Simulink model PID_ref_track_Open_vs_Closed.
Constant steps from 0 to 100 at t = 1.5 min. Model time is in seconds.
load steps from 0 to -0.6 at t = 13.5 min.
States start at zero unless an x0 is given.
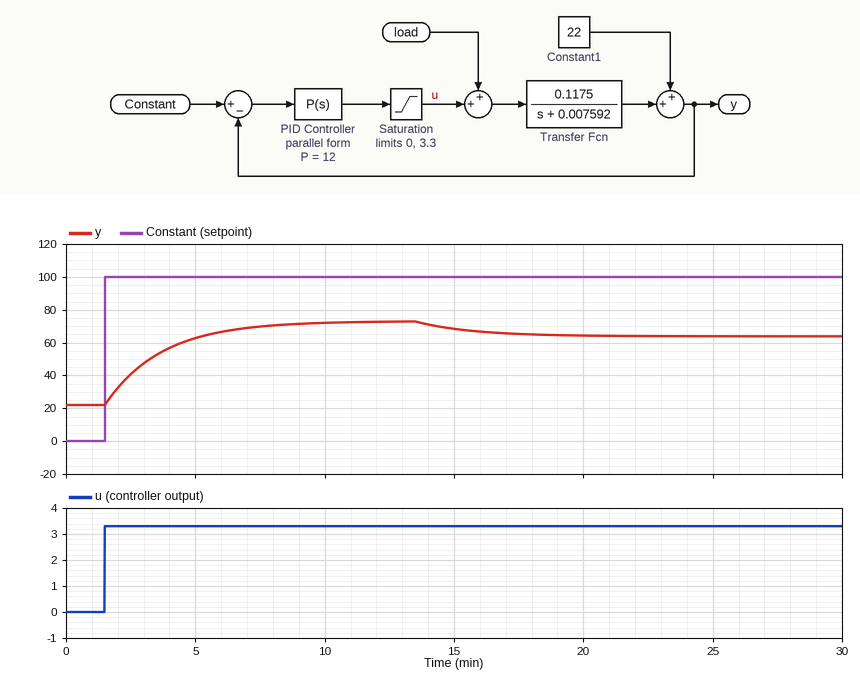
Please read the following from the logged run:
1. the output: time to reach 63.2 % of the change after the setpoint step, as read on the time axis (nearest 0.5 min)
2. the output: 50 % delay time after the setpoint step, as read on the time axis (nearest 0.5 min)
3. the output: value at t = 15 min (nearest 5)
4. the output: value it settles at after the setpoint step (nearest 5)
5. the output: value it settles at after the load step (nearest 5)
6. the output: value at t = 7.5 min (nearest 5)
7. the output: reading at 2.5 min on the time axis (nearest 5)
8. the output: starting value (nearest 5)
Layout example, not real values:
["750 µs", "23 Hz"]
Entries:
["3.5 min", "3.0 min", "70", "75", "65", "70", "40", "20"]
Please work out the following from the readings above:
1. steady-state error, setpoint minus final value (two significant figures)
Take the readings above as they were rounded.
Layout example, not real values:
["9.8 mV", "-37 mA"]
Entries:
["25"]
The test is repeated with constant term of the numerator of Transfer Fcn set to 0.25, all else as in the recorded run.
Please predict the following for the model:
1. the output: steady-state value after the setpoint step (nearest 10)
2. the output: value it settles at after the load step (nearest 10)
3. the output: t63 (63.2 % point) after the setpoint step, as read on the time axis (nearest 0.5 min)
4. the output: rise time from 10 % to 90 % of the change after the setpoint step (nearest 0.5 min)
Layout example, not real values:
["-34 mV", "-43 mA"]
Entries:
["100", "100", "3.0 min", "2.0 min"]
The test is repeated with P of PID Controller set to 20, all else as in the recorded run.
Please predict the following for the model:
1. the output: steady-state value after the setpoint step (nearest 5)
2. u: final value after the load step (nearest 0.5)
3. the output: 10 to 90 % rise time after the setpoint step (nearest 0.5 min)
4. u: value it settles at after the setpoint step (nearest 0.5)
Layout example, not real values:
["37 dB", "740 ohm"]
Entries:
["75", "3.5", "5.0 min", "3.5"]
